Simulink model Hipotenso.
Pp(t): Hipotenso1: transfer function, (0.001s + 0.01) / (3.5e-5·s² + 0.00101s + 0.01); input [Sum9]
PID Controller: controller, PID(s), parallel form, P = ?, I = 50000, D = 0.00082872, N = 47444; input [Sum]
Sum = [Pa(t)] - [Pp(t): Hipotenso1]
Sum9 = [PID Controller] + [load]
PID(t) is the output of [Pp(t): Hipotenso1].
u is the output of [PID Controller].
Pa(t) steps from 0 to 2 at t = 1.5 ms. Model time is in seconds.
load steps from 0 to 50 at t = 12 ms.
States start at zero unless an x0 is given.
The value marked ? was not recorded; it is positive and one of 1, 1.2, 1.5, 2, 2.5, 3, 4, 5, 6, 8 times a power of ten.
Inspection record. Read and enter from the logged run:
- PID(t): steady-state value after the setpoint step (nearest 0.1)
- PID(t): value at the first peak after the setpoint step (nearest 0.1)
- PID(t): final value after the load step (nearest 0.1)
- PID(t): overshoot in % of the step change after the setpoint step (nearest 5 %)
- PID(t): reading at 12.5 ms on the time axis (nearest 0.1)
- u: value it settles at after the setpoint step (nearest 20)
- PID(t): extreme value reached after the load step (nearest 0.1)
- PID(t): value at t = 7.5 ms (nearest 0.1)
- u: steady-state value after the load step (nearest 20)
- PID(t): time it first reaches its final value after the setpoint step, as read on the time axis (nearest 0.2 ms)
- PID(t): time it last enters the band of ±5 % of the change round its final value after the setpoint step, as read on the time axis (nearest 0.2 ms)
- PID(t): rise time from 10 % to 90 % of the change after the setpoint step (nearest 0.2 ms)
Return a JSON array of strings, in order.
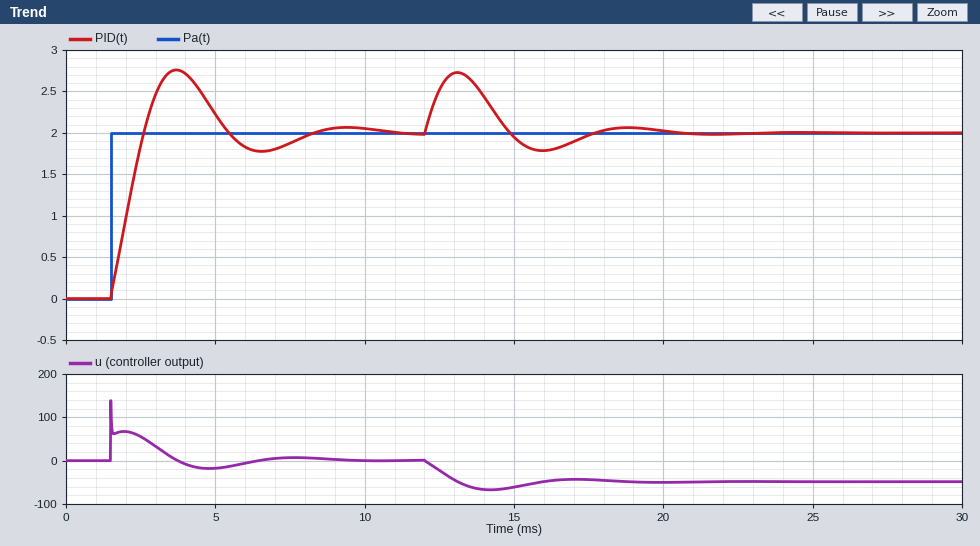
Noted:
["2.0", "2.8", "2.0", "40 %", "2.5", "0", "2.7", "1.9", "-40", "2.6 ms", "7.6 ms", "0.8 ms"]
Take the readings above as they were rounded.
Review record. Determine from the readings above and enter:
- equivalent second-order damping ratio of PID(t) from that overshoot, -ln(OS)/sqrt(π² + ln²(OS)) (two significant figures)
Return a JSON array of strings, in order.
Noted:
["0.28"]
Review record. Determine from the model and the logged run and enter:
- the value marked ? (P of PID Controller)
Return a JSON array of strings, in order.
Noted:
["30"]
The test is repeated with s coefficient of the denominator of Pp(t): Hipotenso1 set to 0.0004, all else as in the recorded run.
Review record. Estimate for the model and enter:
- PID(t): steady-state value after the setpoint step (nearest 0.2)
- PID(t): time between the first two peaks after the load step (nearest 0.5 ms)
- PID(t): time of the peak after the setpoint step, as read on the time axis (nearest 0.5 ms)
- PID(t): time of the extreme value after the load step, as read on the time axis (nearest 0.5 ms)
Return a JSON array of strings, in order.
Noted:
["2.0", "5.5 ms", "3.5 ms", "13.0 ms"]
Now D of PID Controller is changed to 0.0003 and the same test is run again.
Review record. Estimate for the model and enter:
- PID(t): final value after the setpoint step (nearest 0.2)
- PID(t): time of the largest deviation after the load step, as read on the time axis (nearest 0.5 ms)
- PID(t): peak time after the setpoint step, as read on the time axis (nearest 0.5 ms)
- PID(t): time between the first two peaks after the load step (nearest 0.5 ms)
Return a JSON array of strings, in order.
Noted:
["2.0", "13.0 ms", "3.5 ms", "5.5 ms"]
